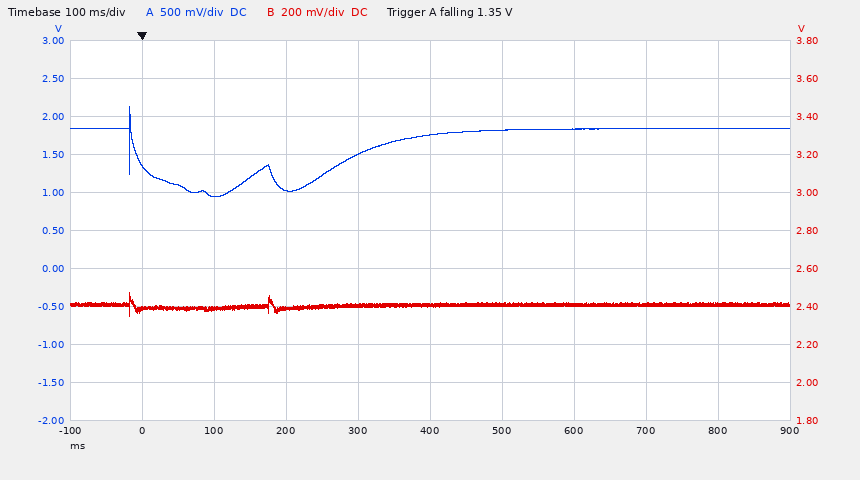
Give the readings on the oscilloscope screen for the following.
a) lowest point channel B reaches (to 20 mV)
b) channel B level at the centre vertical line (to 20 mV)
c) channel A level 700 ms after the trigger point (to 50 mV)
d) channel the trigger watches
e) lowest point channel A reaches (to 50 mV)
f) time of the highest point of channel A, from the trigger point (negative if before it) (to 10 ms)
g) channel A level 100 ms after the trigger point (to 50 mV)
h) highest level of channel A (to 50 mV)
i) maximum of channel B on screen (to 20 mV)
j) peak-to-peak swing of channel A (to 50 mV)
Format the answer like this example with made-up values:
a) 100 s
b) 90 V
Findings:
a) 2.34 V
b) 2.40 V
c) 1.85 V
d) channel A
e) 950 mV
f) -20 ms
g) 950 mV
h) 2.15 V
i) 2.48 V
j) 1.20 V
